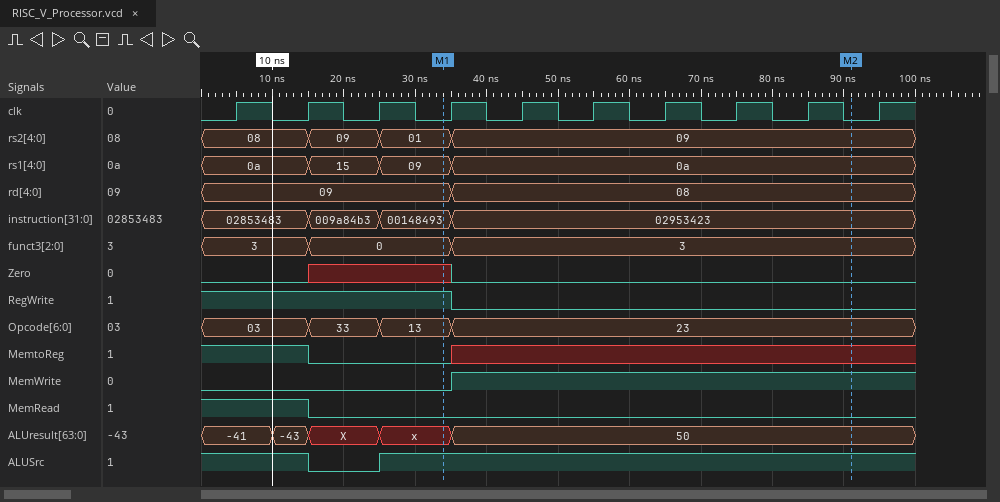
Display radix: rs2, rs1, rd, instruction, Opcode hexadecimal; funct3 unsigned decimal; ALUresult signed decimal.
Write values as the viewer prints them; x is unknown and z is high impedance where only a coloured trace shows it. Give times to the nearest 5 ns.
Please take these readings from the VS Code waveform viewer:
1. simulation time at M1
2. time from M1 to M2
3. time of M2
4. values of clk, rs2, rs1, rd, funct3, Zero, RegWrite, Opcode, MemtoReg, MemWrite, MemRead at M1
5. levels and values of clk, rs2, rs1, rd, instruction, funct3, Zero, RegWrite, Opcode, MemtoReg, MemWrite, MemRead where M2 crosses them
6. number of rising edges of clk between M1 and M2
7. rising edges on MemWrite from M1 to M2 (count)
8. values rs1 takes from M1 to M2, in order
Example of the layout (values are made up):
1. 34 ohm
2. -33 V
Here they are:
1. 35 ns
2. 55 ns
3. 90 ns
4. clk=0, rs2=01, rs1=09, rd=09, funct3=0, Zero=x, RegWrite=1, Opcode=13, MemtoReg=0, MemWrite=0, MemRead=0
5. clk=0, rs2=09, rs1=0a, rd=08, instruction=02953423, funct3=3, Zero=0, RegWrite=0, Opcode=23, MemtoReg=x, MemWrite=1, MemRead=0
6. 6
7. 1
8. 09, 0a
